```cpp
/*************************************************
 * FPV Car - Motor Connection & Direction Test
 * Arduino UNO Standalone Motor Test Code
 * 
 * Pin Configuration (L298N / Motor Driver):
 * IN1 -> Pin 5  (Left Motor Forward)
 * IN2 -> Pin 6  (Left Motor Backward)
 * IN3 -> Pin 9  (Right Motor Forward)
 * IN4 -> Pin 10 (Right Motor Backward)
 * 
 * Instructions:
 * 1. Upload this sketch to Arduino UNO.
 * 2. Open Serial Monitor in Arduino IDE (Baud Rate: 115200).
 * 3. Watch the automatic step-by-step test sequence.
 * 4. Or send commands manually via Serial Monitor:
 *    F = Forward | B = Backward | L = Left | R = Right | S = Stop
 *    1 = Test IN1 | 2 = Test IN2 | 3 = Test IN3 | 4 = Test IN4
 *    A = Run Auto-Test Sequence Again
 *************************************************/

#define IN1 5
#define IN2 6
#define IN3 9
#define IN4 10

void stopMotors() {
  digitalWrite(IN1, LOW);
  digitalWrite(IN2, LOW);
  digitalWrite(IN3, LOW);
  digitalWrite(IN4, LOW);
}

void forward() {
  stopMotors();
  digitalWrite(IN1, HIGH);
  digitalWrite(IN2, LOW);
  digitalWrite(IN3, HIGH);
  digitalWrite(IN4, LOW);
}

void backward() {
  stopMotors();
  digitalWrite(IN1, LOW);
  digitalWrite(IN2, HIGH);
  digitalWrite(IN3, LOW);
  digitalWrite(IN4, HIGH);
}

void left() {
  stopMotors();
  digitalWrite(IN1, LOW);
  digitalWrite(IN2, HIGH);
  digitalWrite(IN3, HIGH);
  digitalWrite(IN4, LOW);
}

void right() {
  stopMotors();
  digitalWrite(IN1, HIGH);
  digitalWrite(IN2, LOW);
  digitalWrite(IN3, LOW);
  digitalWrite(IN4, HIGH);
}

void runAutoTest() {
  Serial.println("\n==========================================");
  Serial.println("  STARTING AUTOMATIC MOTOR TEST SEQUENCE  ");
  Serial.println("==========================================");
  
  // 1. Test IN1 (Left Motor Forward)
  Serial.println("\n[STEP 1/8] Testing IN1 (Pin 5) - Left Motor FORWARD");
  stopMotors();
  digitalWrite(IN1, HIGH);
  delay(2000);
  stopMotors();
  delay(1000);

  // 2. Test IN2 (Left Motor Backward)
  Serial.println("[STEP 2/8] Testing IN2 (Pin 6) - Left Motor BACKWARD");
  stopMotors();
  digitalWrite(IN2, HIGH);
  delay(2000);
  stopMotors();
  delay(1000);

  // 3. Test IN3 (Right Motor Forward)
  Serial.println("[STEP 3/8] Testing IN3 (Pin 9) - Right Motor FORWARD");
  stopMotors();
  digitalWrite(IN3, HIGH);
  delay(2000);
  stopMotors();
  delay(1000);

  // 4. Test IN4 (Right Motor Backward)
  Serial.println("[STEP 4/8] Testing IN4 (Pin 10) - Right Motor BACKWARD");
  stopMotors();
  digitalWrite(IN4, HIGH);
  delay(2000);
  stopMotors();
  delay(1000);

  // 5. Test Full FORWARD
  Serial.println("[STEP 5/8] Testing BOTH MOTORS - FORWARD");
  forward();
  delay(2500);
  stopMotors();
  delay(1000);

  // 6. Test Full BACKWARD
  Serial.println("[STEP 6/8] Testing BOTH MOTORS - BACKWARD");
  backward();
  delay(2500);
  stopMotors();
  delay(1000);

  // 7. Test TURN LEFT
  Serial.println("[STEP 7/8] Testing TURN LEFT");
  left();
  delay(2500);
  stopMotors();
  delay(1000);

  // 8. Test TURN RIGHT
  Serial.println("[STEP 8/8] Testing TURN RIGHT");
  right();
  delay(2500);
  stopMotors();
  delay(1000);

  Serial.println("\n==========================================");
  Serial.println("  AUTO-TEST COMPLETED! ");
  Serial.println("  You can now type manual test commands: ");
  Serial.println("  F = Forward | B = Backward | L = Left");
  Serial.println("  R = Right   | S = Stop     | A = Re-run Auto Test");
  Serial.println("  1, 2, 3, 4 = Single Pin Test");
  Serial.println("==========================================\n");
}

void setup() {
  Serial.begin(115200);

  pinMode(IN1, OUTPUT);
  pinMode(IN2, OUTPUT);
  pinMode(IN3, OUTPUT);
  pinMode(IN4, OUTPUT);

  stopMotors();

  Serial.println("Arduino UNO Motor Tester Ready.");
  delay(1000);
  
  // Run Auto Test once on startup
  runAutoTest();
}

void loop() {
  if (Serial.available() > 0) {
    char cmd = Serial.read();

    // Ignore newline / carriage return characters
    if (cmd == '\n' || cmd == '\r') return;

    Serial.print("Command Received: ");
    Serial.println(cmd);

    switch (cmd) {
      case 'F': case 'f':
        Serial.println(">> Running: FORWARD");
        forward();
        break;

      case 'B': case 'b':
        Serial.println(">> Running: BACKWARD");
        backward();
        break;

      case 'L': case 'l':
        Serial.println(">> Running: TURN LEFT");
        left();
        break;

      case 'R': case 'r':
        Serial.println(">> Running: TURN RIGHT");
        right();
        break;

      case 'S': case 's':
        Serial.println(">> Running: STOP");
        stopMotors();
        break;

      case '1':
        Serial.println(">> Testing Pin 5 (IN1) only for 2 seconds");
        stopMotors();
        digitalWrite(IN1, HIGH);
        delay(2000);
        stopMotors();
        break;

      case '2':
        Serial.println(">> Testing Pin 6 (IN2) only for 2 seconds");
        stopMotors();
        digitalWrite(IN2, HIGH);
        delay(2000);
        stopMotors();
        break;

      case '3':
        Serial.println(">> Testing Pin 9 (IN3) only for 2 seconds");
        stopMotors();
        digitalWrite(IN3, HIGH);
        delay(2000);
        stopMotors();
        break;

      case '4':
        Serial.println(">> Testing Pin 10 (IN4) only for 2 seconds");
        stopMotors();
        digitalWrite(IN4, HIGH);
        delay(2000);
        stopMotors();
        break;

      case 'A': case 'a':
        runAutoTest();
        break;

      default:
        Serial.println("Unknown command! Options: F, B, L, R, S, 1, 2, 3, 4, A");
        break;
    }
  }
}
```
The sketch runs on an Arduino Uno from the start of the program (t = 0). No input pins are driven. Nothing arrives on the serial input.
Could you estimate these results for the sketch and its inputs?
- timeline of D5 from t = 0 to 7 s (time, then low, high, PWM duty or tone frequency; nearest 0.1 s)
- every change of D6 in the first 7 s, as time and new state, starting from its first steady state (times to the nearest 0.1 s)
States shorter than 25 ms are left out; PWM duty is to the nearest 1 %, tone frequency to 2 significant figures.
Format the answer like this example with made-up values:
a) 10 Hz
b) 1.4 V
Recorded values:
a) 0 s low; 1 s high; 3 s low
b) 0 s low; 4 s high; 6 s low
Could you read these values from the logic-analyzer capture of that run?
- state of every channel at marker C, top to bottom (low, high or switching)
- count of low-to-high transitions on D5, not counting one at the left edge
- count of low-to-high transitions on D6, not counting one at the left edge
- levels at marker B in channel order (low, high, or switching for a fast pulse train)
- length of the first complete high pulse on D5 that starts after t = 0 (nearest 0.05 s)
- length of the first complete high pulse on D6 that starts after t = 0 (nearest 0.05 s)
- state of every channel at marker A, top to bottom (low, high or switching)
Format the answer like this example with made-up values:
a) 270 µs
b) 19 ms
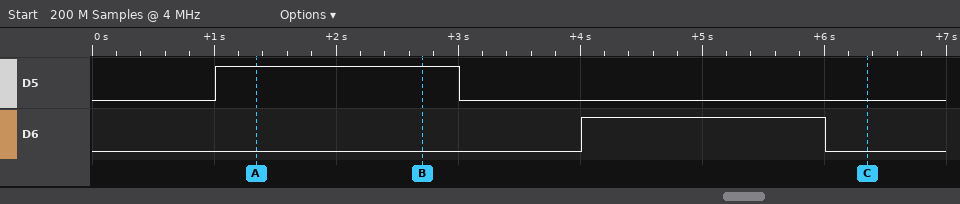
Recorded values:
a) D5 low, D6 low
b) 1
c) 1
d) D5 high, D6 low
e) 2.00 s
f) 2.00 s
g) D5 high, D6 low
